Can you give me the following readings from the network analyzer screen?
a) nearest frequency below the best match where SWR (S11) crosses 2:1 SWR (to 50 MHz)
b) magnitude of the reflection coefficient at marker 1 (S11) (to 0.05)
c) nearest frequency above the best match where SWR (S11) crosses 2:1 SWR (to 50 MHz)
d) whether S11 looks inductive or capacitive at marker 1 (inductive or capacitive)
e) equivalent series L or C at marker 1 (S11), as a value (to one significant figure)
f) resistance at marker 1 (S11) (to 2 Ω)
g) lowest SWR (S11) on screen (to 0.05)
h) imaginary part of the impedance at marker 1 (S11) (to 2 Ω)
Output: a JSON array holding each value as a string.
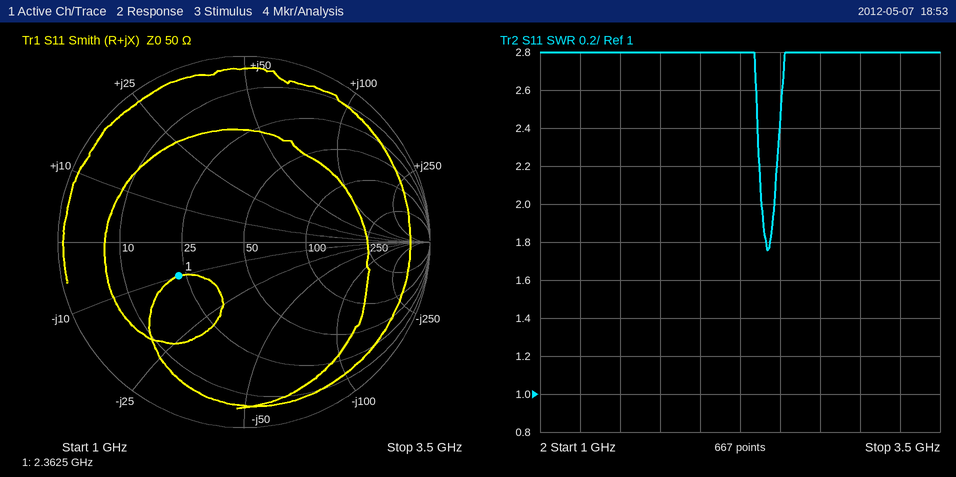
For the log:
["2.40 GHz", "0.40", "2.45 GHz", "capacitive", "7 pF", "22 Ω", "1.75", "-10 Ω"]
